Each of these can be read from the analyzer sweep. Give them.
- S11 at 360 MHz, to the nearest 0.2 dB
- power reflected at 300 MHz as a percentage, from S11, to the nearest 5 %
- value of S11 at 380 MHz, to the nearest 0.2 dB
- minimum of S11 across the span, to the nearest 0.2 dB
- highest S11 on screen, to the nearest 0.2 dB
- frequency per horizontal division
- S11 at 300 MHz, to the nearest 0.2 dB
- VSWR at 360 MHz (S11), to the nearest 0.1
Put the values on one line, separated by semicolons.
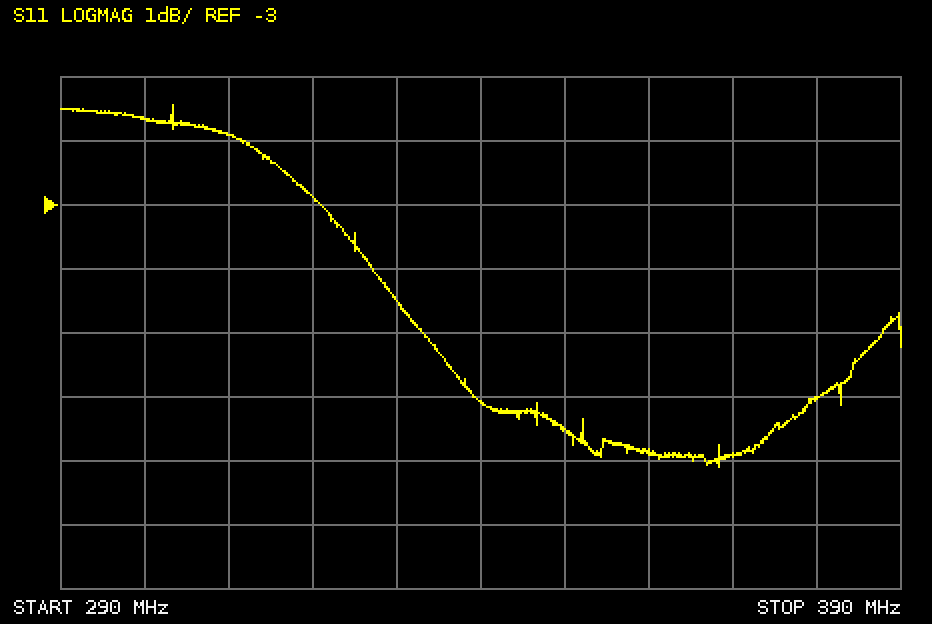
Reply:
-6.8 dB; 70 %; -6.0 dB; -7.0 dB; -1.4 dB; 10 MHz; -1.6 dB; 2.7
